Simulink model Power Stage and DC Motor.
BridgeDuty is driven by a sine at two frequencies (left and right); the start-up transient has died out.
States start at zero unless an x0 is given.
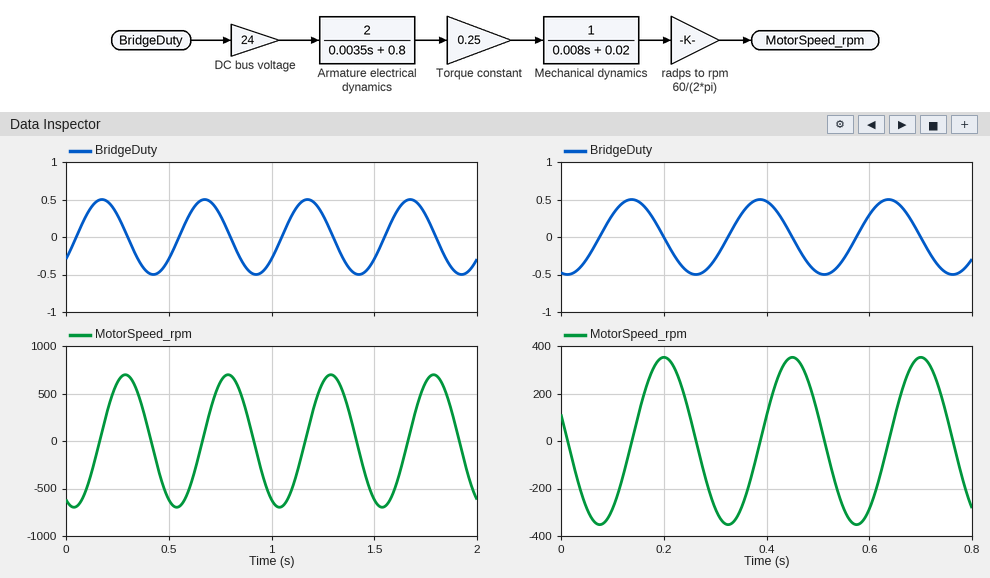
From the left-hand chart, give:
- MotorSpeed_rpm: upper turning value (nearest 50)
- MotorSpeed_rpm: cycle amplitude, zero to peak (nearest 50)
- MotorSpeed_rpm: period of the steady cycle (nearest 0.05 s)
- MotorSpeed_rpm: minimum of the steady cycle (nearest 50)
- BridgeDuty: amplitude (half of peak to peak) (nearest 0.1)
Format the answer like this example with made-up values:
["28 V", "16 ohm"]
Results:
["700", "700", "0.50 s", "-700", "0.5"]
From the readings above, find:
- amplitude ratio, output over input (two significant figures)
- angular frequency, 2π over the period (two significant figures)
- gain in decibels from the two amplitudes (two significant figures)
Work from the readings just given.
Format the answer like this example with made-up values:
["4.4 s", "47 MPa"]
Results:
["1400", "13 rad/s", "63 dB"]
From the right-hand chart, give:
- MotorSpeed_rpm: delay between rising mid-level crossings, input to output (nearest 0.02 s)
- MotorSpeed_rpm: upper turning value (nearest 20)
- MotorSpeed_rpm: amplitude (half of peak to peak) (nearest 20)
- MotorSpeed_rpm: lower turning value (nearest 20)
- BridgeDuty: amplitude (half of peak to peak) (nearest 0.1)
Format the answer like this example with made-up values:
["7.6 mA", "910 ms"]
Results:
["0.06 s", "360", "360", "-360", "0.5"]
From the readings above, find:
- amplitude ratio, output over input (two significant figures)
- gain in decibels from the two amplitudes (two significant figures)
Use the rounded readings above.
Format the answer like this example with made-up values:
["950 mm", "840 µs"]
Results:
["720", "57 dB"]
